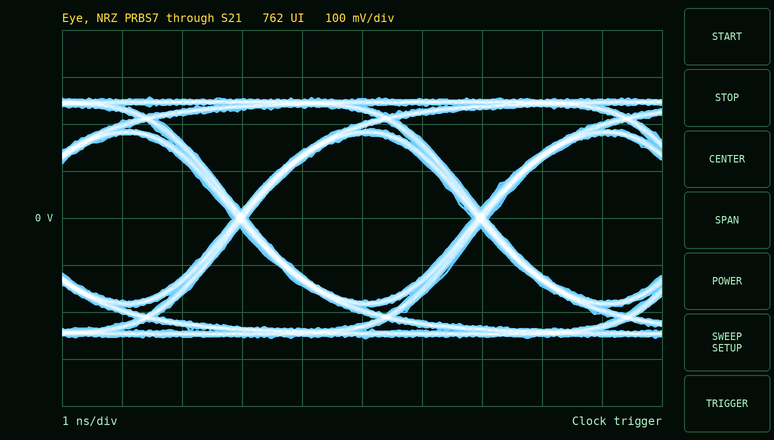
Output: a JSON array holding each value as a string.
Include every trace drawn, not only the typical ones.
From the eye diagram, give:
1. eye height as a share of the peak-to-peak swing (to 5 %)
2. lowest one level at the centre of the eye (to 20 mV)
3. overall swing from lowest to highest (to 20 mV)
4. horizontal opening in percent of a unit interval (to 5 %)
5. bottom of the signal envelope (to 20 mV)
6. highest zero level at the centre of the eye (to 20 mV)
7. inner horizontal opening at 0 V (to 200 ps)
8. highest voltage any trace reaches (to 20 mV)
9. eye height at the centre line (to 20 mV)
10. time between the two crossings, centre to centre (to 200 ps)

["70 %", "180 mV", "520 mV", "95 %", "-260 mV", "-180 mV", "3.8 ns", "260 mV", "360 mV", "4.0 ns"]
